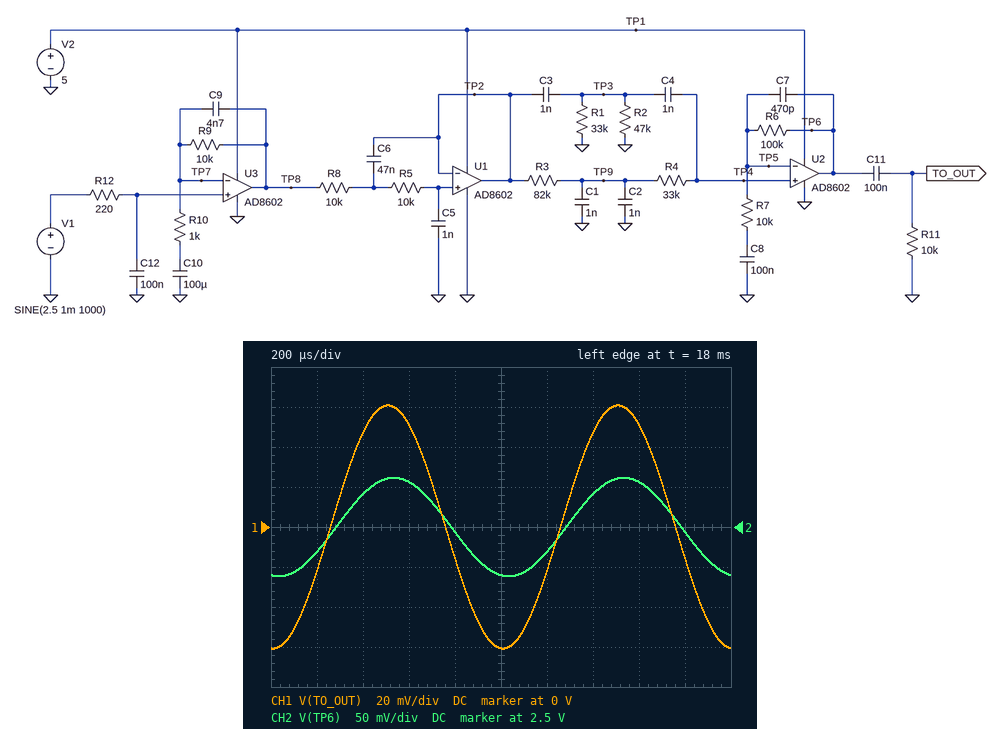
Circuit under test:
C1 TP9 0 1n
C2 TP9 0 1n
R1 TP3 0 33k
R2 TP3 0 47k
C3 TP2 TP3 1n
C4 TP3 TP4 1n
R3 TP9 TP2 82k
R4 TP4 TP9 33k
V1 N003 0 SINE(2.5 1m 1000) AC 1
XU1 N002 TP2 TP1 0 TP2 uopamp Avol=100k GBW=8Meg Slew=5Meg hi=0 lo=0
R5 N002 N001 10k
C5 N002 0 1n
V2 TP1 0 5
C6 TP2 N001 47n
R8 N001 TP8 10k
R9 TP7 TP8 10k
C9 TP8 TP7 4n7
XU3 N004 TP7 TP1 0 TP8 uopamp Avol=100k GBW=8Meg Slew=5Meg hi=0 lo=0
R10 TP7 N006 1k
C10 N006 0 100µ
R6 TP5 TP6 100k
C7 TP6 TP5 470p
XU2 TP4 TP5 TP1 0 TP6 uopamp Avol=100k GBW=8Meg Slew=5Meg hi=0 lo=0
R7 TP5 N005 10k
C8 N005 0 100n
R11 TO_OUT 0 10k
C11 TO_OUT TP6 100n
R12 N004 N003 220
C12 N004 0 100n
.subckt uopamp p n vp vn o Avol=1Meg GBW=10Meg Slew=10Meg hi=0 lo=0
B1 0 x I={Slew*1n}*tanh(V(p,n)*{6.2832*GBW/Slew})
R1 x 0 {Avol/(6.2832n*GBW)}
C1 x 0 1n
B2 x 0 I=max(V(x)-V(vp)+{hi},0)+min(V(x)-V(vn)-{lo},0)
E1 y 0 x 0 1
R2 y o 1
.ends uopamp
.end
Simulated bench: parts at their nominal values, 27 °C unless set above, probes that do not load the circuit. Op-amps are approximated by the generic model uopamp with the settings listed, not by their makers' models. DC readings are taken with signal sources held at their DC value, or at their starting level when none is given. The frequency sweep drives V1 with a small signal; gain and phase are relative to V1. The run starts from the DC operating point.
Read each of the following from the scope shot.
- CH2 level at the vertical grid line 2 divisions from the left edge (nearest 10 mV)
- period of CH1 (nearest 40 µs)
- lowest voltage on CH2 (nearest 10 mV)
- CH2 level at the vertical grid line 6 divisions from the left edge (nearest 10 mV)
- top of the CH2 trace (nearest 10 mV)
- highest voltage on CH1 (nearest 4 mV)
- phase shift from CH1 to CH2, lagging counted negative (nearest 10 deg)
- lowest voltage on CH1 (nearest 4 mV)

2.54 V
1.00 ms
2.44 V
2.47 V
2.56 V
60 mV
-10 deg
-60 mV
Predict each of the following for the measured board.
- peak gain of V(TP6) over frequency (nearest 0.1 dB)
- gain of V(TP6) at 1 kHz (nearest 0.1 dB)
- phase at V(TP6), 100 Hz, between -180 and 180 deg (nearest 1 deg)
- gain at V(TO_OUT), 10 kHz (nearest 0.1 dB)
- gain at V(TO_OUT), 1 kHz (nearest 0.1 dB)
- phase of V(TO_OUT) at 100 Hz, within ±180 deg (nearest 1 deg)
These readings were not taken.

39.6 dB
35.8 dB
36 deg
-13.9 dB
35.7 dB
94 deg
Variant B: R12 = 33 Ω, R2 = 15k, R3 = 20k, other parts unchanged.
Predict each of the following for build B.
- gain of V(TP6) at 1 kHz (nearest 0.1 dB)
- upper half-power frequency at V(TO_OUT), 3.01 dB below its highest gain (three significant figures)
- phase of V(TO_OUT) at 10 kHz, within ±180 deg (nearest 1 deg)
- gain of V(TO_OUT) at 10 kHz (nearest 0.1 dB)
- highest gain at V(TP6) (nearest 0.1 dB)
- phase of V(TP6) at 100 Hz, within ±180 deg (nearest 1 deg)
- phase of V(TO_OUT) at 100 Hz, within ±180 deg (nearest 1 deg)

41.3 dB
2.48 kHz
143 deg
-15.4 dB
44.5 dB
43 deg
101 deg
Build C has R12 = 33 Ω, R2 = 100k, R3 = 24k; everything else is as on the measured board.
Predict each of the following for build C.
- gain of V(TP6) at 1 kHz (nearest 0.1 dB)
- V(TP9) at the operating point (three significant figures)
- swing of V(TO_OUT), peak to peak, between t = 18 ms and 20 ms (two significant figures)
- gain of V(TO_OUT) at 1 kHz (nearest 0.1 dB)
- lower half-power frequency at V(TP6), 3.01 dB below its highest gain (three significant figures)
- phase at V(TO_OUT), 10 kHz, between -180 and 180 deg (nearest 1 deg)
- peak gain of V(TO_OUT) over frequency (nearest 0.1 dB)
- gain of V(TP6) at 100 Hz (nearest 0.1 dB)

40.6 dB
2.50 V
210 mV
40.5 dB
199 Hz
116 deg
42.5 dB
36.3 dB
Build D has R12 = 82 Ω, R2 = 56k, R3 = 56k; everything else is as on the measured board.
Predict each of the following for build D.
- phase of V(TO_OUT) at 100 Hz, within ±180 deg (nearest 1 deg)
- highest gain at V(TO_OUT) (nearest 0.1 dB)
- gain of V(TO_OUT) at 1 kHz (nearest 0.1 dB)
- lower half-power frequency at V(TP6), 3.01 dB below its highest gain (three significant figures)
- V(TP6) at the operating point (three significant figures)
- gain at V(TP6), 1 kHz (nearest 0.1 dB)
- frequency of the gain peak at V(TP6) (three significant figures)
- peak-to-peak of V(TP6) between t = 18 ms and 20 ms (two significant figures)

97 deg
39.6 dB
37.9 dB
118 Hz
2.50 V
38.0 dB
366 Hz
160 mV
